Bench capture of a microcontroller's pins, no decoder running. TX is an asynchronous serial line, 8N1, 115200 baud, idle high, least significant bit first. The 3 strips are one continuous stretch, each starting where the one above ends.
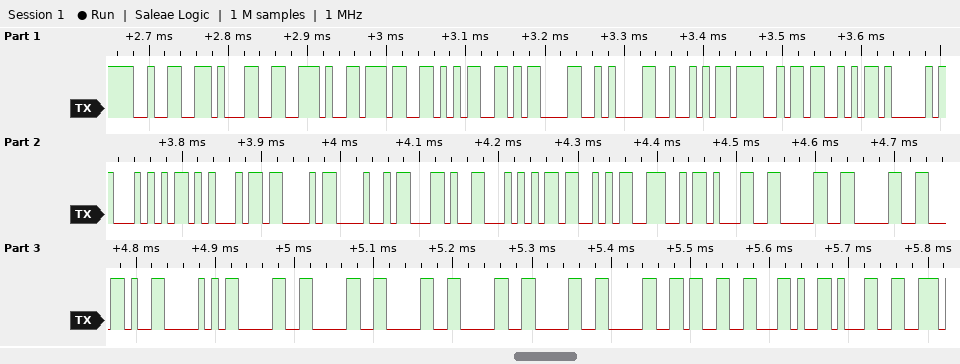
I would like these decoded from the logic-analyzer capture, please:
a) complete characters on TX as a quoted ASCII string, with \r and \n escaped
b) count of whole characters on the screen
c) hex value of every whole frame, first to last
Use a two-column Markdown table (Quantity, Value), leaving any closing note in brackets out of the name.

| Quantity | Value |
|---|---|
| complete characters on TX as a quoted ASCII string, with \r and \n escaped | "21.75\r\nROSATECH,TSN100,P0000003,1" |
| count of whole characters on the screen | 33 |
| hex value of every whole frame, first to last | 32 31 2E 37 35 0D 0A 52 4F 53 41 54 45 43 48 2C 54 53 4E 31 30 30 2C 50 30 30 30 30 30 30 33 2C 31 |
